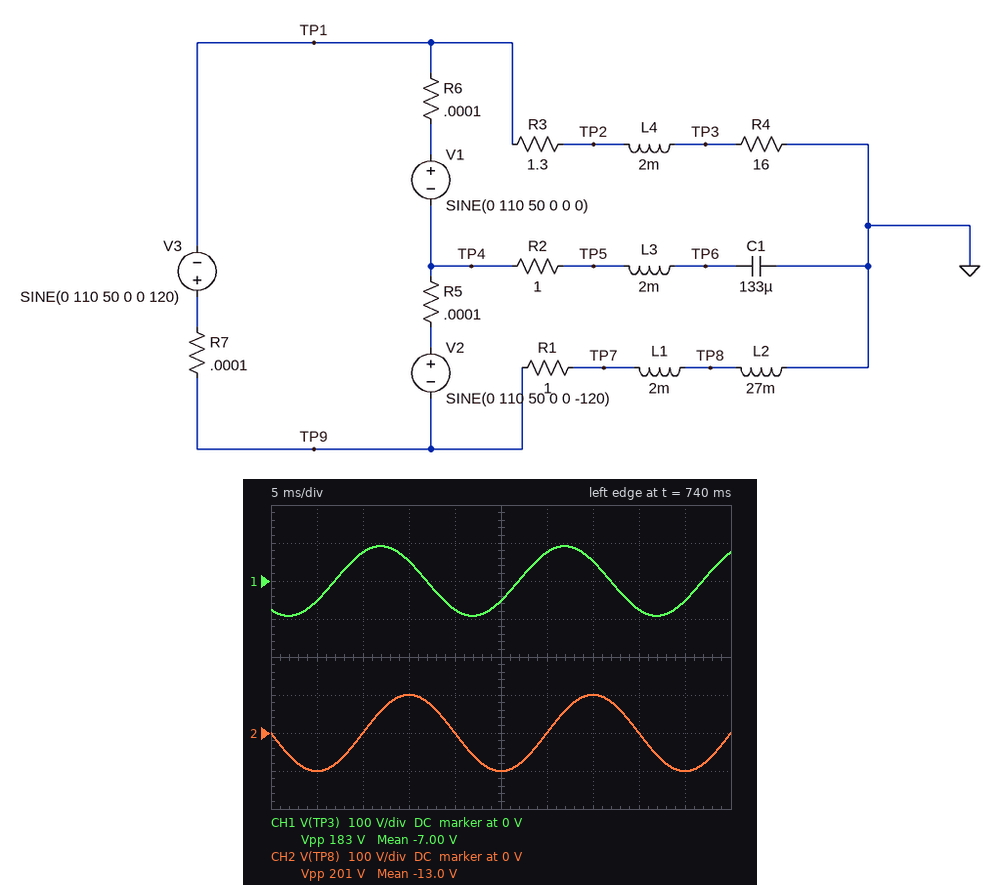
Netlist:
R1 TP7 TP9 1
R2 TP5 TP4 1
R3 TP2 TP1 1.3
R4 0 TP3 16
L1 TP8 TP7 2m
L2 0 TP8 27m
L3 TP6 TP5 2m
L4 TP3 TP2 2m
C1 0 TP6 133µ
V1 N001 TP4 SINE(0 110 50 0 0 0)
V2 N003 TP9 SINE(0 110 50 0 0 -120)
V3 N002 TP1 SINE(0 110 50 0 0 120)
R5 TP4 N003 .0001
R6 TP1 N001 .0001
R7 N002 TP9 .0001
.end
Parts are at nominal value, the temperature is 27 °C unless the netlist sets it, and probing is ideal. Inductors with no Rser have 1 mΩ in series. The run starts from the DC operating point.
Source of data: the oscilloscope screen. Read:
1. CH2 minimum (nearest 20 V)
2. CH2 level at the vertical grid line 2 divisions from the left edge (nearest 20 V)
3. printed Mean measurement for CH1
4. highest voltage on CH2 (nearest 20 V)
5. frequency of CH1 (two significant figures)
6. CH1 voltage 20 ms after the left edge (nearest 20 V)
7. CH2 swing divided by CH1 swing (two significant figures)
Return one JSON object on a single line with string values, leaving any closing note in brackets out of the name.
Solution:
{"CH2 minimum": "-100 V", "CH2 level at the vertical grid line 2 divisions from the left edge": "0 V", "printed Mean measurement for CH1": "-7.00 V", "highest voltage on CH2": "100 V", "frequency of CH1": "50 Hz", "CH1 voltage 20 ms after the left edge": "-80 V", "CH2 swing divided by CH1 swing": "1.1"}
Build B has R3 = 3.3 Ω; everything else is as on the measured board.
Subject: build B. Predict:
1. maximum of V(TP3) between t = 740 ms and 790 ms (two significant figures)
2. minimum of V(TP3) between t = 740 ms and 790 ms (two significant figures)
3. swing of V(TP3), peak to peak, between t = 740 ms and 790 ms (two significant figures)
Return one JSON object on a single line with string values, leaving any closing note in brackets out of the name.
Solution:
{"maximum of V(TP3) between t = 740 ms and 790 ms": "86 V", "minimum of V(TP3) between t = 740 ms and 790 ms": "-86 V", "swing of V(TP3), peak to peak, between t = 740 ms and 790 ms": "170 V"}
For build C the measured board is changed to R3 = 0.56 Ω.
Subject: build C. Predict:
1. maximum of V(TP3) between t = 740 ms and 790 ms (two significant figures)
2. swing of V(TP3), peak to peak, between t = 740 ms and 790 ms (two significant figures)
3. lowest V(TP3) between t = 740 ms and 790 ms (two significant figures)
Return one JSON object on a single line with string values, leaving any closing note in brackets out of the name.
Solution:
{"maximum of V(TP3) between t = 740 ms and 790 ms": "94 V", "swing of V(TP3), peak to peak, between t = 740 ms and 790 ms": "190 V", "lowest V(TP3) between t = 740 ms and 790 ms": "-94 V"}
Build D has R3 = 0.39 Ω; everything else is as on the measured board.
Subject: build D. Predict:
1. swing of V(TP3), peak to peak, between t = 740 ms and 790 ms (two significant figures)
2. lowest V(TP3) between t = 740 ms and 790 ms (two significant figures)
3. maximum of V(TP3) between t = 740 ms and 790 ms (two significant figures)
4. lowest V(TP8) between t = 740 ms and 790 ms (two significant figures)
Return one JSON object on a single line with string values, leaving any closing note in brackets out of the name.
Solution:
{"swing of V(TP3), peak to peak, between t = 740 ms and 790 ms": "190 V", "lowest V(TP3) between t = 740 ms and 790 ms": "-94 V", "maximum of V(TP3) between t = 740 ms and 790 ms": "94 V", "lowest V(TP8) between t = 740 ms and 790 ms": "-100 V"}
